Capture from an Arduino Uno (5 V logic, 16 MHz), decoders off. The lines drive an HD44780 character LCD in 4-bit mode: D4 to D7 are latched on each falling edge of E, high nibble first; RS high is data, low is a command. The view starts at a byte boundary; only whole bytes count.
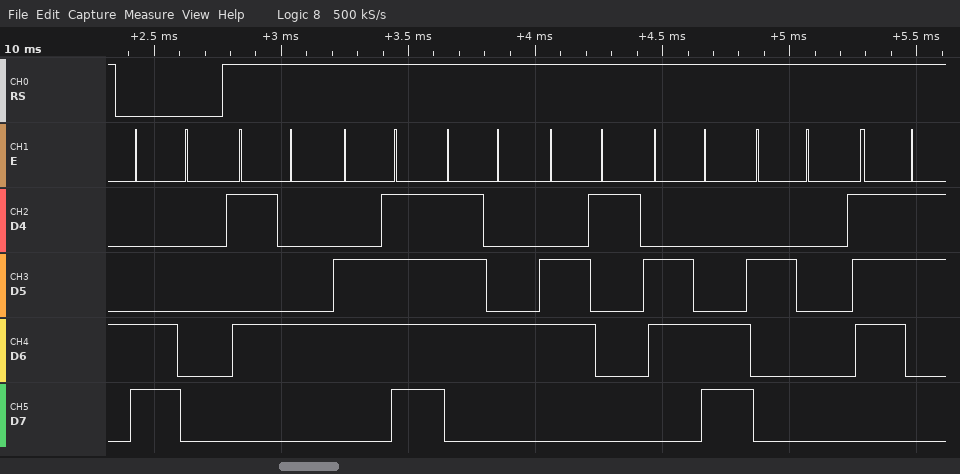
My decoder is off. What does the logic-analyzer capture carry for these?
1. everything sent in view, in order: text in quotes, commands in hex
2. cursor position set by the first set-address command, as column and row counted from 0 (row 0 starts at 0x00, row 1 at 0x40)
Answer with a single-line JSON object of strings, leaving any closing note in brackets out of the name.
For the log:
{"everything sent in view, in order: text in quotes, commands in hex": "0xC0 \"Total s\"", "cursor position set by the first set-address command, as column and row counted from 0": "column 0, row 1"}
